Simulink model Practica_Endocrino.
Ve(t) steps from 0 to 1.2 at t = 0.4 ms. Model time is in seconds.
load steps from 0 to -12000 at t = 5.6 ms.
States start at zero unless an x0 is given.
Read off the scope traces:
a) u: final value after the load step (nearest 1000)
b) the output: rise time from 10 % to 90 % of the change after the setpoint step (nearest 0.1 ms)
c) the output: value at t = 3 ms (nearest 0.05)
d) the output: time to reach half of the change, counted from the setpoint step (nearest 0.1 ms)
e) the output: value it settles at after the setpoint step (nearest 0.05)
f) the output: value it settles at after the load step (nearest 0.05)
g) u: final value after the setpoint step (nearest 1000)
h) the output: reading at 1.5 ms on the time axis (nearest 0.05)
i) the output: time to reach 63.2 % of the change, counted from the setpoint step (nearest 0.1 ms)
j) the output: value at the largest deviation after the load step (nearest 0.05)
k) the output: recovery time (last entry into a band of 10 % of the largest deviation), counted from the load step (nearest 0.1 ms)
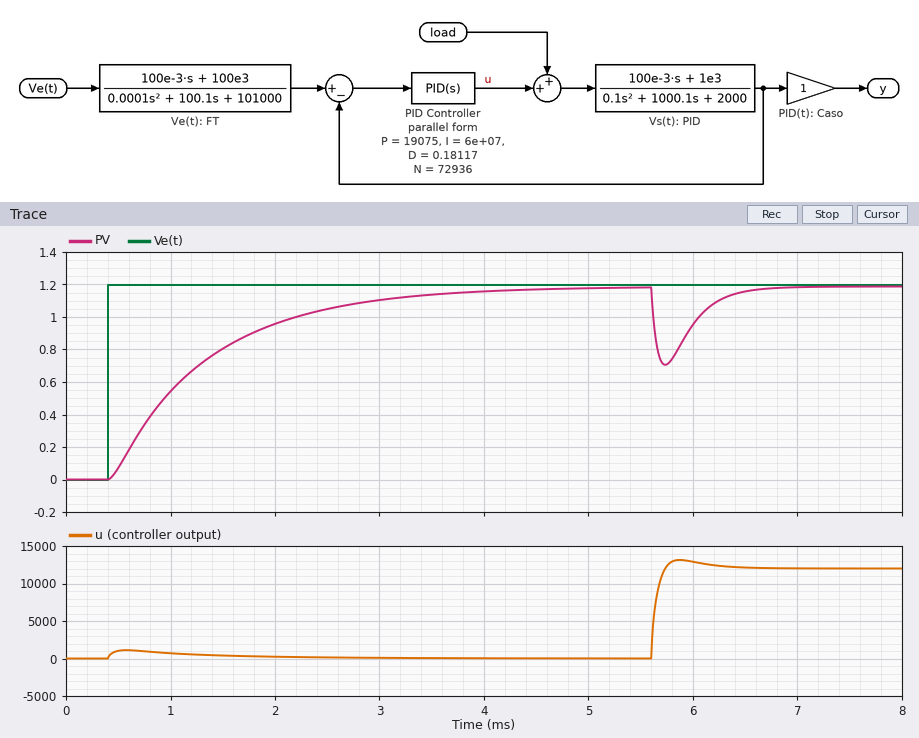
12000
2.1 ms
1.10
0.7 ms
1.20
1.20
0
0.80
1.0 ms
0.70
0.8 ms
